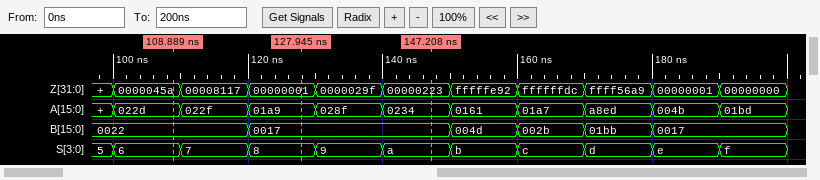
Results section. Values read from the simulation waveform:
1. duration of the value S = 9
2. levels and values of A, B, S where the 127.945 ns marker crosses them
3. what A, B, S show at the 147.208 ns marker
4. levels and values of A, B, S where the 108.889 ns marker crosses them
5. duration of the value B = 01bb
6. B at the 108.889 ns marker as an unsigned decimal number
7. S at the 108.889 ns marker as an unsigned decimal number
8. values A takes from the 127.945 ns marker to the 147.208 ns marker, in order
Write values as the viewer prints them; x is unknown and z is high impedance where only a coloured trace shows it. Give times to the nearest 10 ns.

10 ns
A=01a9, B=0017, S=8
A=0234, B=0017, S=a
A=022d, B=0022, S=6
10 ns
34
6
01a9, 028f, 0234
